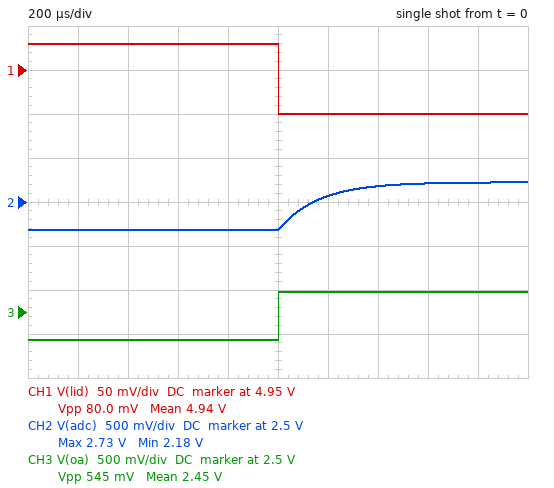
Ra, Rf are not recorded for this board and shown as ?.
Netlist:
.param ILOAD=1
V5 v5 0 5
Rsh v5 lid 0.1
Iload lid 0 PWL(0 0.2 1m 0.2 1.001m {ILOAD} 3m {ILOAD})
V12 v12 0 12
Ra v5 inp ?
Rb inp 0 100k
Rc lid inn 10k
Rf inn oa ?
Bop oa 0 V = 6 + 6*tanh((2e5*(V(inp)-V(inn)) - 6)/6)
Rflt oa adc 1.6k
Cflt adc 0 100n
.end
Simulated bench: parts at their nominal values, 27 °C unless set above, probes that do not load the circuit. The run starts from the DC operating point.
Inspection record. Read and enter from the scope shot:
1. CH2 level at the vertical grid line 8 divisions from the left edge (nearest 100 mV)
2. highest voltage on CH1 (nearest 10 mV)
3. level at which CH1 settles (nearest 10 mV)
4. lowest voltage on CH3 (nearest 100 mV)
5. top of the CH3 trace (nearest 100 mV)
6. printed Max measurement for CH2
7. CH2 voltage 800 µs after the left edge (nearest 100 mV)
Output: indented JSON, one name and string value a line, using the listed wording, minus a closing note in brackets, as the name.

{
  "CH2 level at the vertical grid line 8 divisions from the left edge": "2.7 V",
  "highest voltage on CH1": "4.98 V",
  "level at which CH1 settles": "4.90 V",
  "lowest voltage on CH3": "2.2 V",
  "top of the CH3 trace": "2.7 V",
  "printed Max measurement for CH2": "2.73 V",
  "CH2 voltage 800 µs after the left edge": "2.2 V"
}
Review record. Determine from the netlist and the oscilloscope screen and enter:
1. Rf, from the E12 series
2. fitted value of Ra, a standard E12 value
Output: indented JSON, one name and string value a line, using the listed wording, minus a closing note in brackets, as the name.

{
  "Rf, from the E12 series": "68 kΩ",
  "fitted value of Ra, a standard E12 value": "8.2 kΩ"
}
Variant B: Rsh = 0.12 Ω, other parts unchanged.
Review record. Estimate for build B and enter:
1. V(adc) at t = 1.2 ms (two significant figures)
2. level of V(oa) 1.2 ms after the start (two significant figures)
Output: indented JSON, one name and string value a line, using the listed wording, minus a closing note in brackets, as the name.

{
  "V(adc) at t = 1.2 ms": "2.7 V",
  "level of V(oa) 1.2 ms after the start": "2.9 V"
}
